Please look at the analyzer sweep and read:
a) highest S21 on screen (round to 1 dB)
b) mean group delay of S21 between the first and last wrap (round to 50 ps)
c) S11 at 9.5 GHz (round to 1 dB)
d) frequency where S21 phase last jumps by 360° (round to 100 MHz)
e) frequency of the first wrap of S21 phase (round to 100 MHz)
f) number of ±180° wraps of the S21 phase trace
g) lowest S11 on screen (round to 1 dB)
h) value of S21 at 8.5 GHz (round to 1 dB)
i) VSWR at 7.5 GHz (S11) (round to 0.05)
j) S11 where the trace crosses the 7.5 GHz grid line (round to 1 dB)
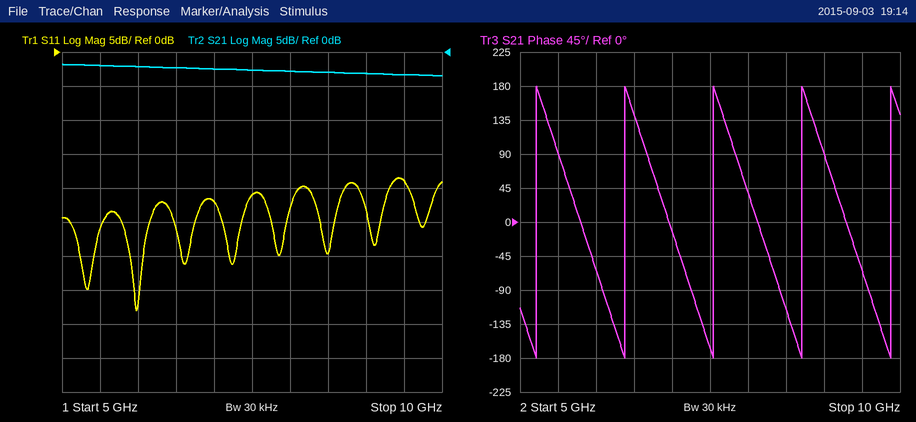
-2 dB
850 ps
-19 dB
9.9 GHz
5.2 GHz
5
-38 dB
-3 dB
1.20
-21 dB
